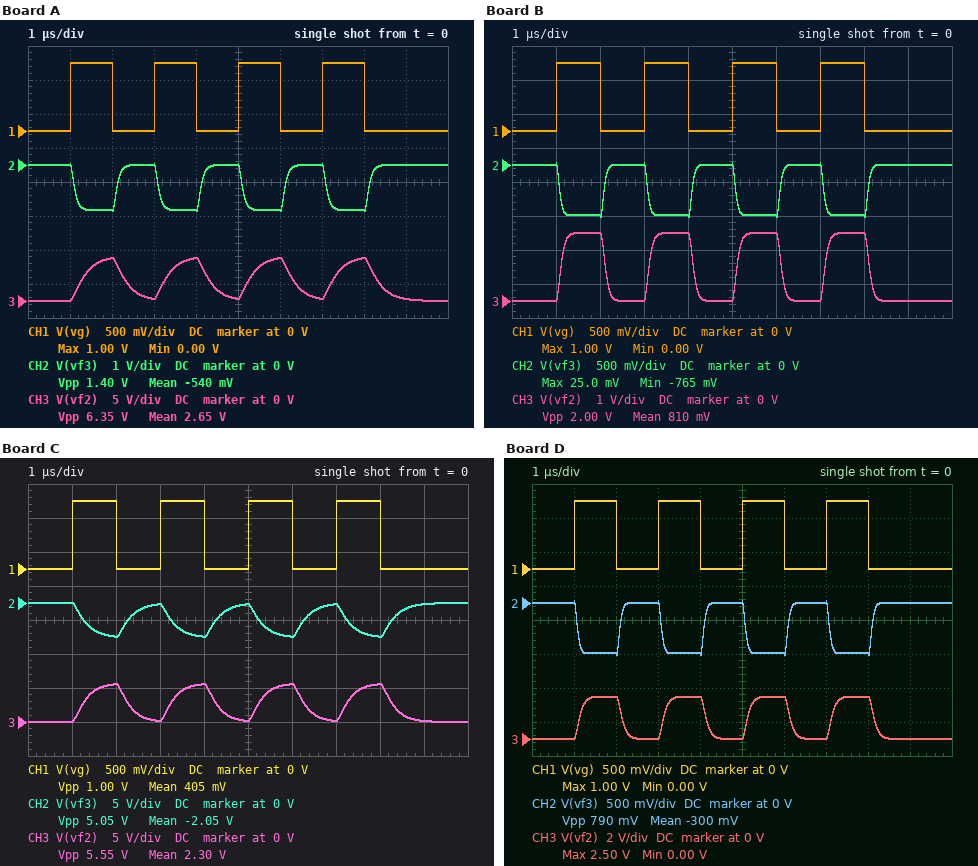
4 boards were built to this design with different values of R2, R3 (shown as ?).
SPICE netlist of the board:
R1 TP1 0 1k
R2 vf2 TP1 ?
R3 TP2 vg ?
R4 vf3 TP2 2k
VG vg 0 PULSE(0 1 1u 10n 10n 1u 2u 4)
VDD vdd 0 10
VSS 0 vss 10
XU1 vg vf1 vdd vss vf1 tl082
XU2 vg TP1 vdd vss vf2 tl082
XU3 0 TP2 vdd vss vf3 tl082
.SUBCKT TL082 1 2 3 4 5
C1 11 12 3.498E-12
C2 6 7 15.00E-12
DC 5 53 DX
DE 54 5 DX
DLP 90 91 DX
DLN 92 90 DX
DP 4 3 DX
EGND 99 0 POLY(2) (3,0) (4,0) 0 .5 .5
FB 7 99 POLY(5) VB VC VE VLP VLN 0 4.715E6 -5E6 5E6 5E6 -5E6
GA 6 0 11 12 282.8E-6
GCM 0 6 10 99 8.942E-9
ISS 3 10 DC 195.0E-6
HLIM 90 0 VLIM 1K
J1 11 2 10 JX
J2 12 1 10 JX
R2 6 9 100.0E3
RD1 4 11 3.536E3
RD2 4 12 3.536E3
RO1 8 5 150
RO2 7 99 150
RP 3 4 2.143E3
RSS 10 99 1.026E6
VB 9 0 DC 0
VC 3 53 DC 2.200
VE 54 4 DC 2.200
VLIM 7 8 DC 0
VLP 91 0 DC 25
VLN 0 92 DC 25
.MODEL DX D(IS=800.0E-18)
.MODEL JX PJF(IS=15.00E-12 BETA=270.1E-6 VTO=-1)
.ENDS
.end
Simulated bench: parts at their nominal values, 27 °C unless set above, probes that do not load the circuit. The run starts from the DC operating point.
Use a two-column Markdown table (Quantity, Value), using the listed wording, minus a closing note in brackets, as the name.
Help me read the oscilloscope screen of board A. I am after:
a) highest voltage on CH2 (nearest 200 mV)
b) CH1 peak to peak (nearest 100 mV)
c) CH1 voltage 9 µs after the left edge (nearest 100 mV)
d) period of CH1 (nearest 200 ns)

| Quantity | Value |
|---|---|
| highest voltage on CH2 | 0 V |
| CH1 peak to peak | 1.0 V |
| CH1 voltage 9 µs after the left edge | 0 V |
| period of CH1 | 2.0 µs |
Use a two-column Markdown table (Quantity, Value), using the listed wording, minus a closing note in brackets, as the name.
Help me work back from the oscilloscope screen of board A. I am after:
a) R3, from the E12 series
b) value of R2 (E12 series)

| Quantity | Value |
|---|---|
| R3, from the E12 series | 1.5 kΩ |
| value of R2 | 5.6 kΩ |
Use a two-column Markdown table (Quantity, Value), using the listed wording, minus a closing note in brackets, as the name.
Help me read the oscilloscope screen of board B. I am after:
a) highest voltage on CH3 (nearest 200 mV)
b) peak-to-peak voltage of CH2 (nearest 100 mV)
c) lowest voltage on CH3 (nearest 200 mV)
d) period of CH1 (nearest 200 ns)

| Quantity | Value |
|---|---|
| highest voltage on CH3 | 2.0 V |
| peak-to-peak voltage of CH2 | 800 mV |
| lowest voltage on CH3 | 0 V |
| period of CH1 | 2.0 µs |
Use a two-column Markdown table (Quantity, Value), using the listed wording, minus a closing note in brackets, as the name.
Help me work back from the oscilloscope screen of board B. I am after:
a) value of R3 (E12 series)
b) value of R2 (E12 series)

| Quantity | Value |
|---|---|
| value of R3 | 2.7 kΩ |
| value of R2 | 1 kΩ |
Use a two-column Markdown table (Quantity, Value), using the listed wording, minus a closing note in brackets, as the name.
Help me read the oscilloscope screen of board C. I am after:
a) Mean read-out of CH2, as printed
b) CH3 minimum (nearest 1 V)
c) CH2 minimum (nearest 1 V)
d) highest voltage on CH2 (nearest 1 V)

| Quantity | Value |
|---|---|
| Mean read-out of CH2, as printed | -2.05 V |
| CH3 minimum | 0 V |
| CH2 minimum | -5 V |
| highest voltage on CH2 | 0 V |
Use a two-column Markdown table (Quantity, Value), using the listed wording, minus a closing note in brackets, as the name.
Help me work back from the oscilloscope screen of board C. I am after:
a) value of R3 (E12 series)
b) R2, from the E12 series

| Quantity | Value |
|---|---|
| value of R3 | 390 Ω |
| R2, from the E12 series | 4.7 kΩ |
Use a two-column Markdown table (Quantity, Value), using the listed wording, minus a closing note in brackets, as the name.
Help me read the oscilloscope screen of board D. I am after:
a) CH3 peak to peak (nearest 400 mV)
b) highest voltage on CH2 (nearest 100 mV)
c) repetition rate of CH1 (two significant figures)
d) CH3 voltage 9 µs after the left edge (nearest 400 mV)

| Quantity | Value |
|---|---|
| CH3 peak to peak | 2.4 V |
| highest voltage on CH2 | 0 V |
| repetition rate of CH1 | 500 kHz |
| CH3 voltage 9 µs after the left edge | 0 V |
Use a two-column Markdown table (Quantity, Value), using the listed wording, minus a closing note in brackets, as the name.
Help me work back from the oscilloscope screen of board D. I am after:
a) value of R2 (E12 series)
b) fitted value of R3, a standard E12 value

| Quantity | Value |
|---|---|
| value of R2 | 1.5 kΩ |
| fitted value of R3, a standard E12 value | 2.7 kΩ |
